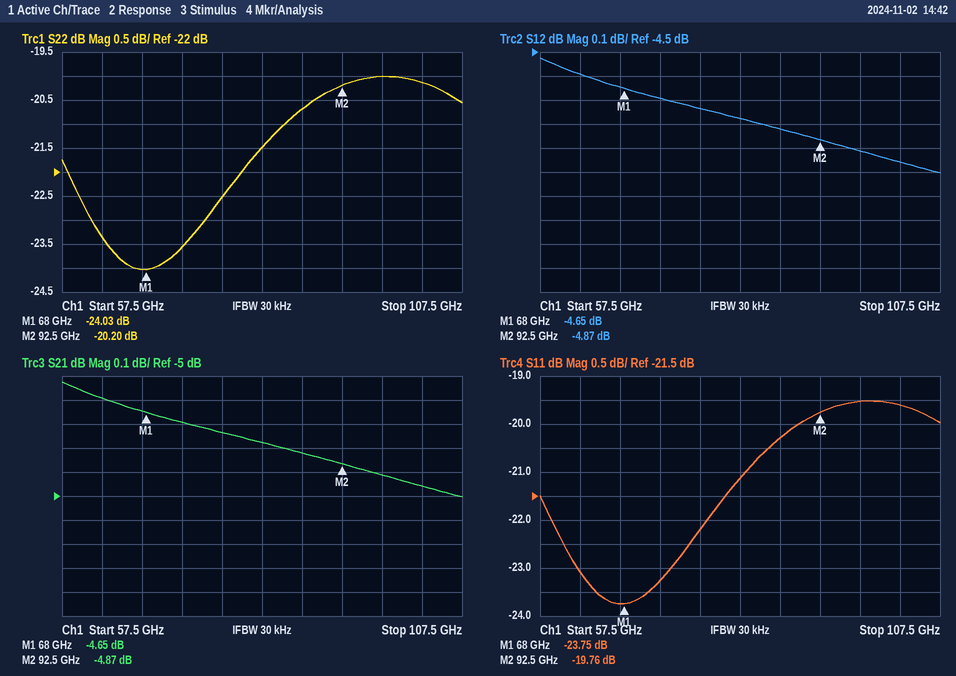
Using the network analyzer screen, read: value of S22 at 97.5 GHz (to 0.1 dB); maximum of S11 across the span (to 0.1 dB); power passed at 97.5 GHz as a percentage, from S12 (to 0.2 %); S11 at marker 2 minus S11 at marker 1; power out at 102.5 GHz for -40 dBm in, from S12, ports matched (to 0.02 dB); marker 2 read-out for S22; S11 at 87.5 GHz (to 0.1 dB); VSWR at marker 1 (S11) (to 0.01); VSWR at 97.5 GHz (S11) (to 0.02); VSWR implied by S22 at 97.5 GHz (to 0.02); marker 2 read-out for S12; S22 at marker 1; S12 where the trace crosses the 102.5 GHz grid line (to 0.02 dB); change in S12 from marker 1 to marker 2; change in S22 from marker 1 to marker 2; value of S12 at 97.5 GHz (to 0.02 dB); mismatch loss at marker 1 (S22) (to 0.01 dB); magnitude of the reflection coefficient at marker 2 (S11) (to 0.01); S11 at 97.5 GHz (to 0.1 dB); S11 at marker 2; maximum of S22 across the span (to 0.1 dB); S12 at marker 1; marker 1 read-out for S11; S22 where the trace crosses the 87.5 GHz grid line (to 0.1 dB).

-20.0 dB
-19.5 dB
32.2 %
3.99 dB
-44.96 dBm
-20.20 dB
-20.3 dB
1.14
1.24
1.22
-4.87 dB
-24.03 dB
-4.96 dB
-0.22 dB
3.83 dB
-4.92 dB
0.02 dB
0.10
-19.5 dB
-19.76 dB
-20.0 dB
-4.65 dB
-23.75 dB
-20.7 dB
